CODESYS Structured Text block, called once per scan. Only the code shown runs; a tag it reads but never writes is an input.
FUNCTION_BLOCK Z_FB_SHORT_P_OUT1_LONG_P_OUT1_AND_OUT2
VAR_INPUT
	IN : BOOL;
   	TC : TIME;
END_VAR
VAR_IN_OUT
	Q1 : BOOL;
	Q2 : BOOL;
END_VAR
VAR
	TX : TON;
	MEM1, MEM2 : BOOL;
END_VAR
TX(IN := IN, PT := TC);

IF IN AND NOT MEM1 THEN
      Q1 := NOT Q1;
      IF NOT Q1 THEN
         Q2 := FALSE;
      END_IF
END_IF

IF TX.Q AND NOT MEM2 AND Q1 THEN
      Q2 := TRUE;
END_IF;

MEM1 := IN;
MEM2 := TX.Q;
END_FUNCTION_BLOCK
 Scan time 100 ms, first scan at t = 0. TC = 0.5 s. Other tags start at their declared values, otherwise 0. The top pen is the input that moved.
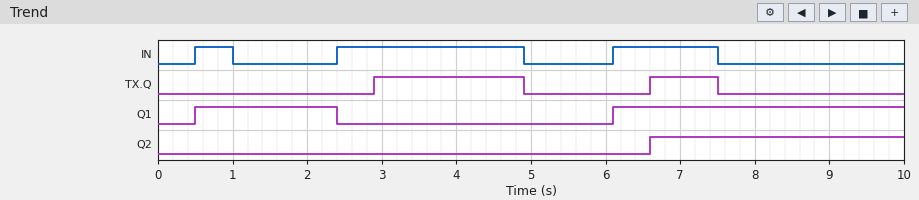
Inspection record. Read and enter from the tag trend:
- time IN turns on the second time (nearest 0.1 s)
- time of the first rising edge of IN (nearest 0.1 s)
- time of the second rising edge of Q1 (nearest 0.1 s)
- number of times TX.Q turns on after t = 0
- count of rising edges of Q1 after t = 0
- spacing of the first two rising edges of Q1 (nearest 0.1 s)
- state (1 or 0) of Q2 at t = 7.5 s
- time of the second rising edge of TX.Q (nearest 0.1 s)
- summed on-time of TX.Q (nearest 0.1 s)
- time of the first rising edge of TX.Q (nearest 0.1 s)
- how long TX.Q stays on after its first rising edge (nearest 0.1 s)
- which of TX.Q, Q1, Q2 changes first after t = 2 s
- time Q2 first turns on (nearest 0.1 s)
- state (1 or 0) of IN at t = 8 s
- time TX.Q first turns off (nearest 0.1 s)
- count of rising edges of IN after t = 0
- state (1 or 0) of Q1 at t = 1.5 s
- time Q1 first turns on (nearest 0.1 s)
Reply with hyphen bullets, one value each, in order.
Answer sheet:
- 2.4 s
- 0.5 s
- 6.1 s
- 2
- 2
- 5.6 s
- 1
- 6.6 s
- 2.9 s
- 2.9 s
- 2.0 s
- Q1
- 6.6 s
- 0
- 4.9 s
- 3
- 1
- 0.5 s
